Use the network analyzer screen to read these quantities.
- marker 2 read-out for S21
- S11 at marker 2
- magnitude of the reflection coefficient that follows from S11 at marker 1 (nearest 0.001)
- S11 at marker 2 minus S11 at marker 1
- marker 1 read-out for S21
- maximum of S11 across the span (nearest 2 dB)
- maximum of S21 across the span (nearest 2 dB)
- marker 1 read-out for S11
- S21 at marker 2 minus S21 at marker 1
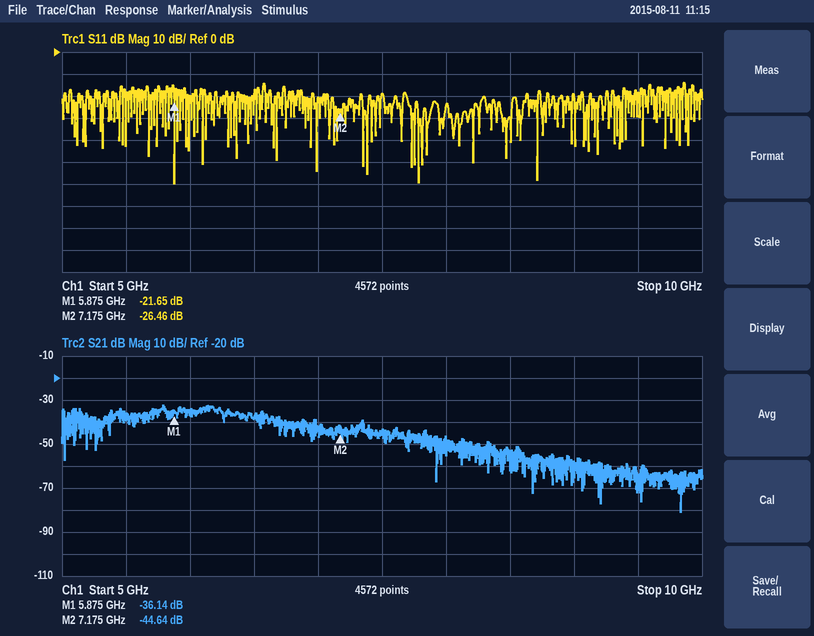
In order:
-44.64 dB
-26.46 dB
0.083
-4.81 dB
-36.14 dB
-14 dB
-32 dB
-21.65 dB
-8.50 dB
